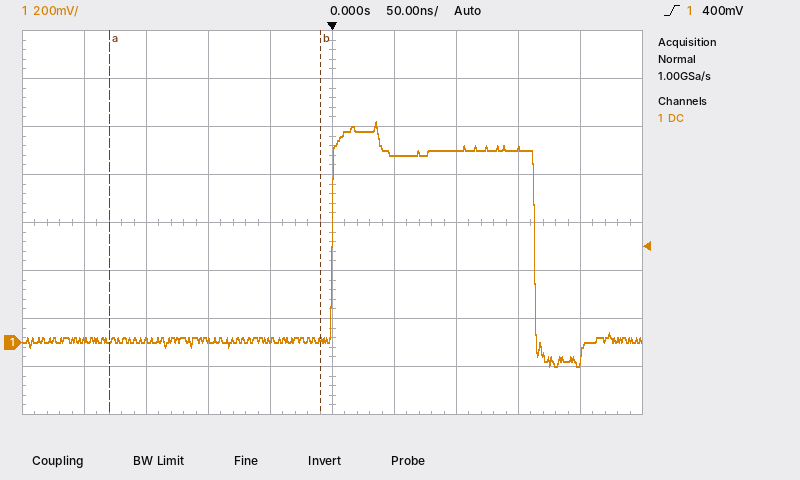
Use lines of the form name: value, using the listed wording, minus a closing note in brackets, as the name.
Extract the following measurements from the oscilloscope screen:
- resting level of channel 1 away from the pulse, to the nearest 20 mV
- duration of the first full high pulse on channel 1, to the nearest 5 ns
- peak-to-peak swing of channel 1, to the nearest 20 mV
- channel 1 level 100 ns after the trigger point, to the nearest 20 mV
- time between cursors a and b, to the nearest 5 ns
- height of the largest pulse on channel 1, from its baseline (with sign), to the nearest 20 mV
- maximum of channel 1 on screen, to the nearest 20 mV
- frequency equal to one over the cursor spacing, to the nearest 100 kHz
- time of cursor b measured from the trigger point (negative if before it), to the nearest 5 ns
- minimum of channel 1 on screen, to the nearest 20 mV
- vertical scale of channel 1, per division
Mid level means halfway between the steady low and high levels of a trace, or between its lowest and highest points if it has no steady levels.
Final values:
resting level of channel 1 away from the pulse, to the nearest 20 mV: 0 mV
duration of the first full high pulse on channel 1, to the nearest 5 ns: 165 ns
peak-to-peak swing of channel 1, to the nearest 20 mV: 1.02 V
channel 1 level 100 ns after the trigger point, to the nearest 20 mV: 800 mV
time between cursors a and b, to the nearest 5 ns: 170 ns
height of the largest pulse on channel 1, from its baseline (with sign), to the nearest 20 mV: +920 mV
maximum of channel 1 on screen, to the nearest 20 mV: 920 mV
frequency equal to one over the cursor spacing, to the nearest 100 kHz: 5.9 MHz
time of cursor b measured from the trigger point (negative if before it), to the nearest 5 ns: -10 ns
minimum of channel 1 on screen, to the nearest 20 mV: -100 mV
vertical scale of channel 1, per division: 200 mV
